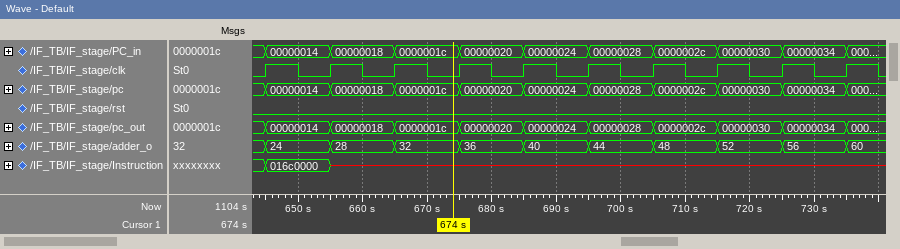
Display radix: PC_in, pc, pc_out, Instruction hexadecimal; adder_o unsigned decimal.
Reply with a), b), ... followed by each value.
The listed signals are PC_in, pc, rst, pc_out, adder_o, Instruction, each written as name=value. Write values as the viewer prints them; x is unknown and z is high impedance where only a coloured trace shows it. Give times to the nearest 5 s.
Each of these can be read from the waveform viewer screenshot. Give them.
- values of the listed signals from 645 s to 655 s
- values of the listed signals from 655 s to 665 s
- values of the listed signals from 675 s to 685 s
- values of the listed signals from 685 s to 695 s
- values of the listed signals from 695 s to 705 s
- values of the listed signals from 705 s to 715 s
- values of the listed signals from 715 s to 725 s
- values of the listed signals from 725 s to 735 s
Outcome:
a) PC_in=00000014, pc=00000014, rst=0, pc_out=00000014, adder_o=24, Instruction=016c0000
b) PC_in=00000018, pc=00000018, rst=0, pc_out=00000018, adder_o=28, Instruction=x
c) PC_in=00000020, pc=00000020, rst=0, pc_out=00000020, adder_o=36, Instruction=x
d) PC_in=00000024, pc=00000024, rst=0, pc_out=00000024, adder_o=40, Instruction=x
e) PC_in=00000028, pc=00000028, rst=0, pc_out=00000028, adder_o=44, Instruction=x
f) PC_in=0000002c, pc=0000002c, rst=0, pc_out=0000002c, adder_o=48, Instruction=x
g) PC_in=00000030, pc=00000030, rst=0, pc_out=00000030, adder_o=52, Instruction=x
h) PC_in=00000034, pc=00000034, rst=0, pc_out=00000034, adder_o=56, Instruction=x
